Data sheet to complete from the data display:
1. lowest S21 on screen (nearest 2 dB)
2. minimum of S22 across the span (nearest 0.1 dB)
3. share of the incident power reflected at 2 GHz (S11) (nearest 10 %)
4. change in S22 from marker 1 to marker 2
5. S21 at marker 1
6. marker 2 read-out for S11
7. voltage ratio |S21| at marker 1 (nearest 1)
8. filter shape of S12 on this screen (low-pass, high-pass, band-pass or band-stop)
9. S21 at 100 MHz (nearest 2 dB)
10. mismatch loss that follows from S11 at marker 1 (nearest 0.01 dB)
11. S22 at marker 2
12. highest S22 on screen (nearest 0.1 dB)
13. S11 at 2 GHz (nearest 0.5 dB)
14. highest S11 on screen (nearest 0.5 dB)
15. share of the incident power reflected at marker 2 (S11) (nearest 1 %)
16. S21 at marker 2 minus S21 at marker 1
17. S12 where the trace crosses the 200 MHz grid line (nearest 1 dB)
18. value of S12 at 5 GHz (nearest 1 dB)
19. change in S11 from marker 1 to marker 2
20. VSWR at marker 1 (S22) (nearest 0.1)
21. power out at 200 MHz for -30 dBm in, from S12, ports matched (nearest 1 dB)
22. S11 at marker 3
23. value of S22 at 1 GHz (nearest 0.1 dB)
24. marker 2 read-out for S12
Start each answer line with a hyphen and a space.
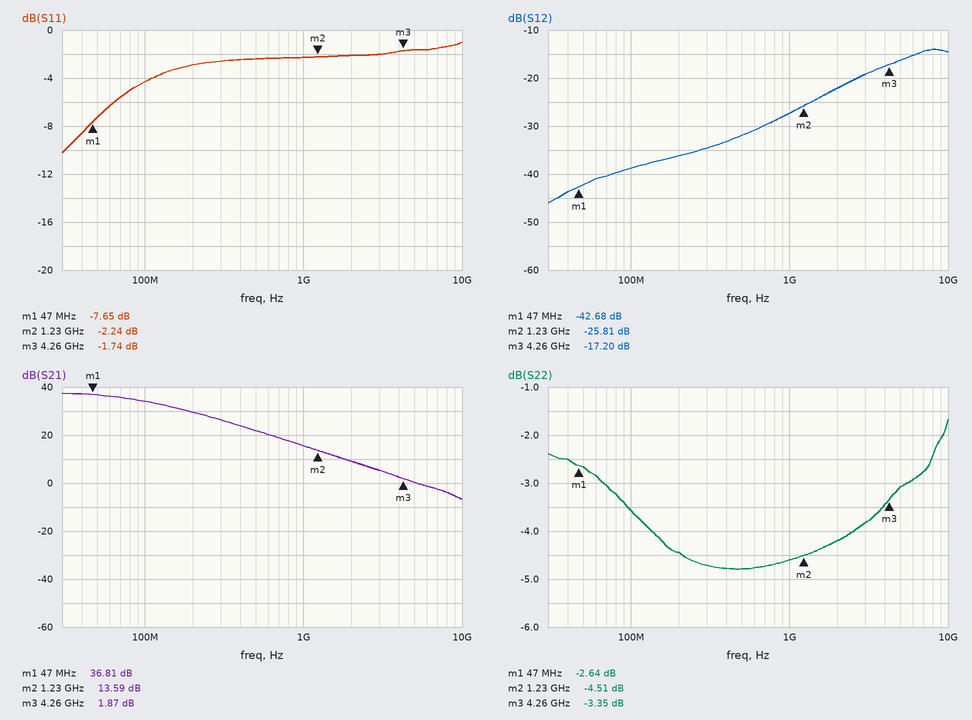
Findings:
- -6 dB
- -4.8 dB
- 60 %
- -1.87 dB
- 36.81 dB
- -2.24 dB
- 69
- high-pass
- 34 dB
- 0.82 dB
- -4.51 dB
- -1.7 dB
- -2.0 dB
- -1.0 dB
- 60 %
- -23.22 dB
- -36 dB
- -16 dB
- 5.41 dB
- 6.6
- -66 dBm
- -1.74 dB
- -4.6 dB
- -25.81 dB
